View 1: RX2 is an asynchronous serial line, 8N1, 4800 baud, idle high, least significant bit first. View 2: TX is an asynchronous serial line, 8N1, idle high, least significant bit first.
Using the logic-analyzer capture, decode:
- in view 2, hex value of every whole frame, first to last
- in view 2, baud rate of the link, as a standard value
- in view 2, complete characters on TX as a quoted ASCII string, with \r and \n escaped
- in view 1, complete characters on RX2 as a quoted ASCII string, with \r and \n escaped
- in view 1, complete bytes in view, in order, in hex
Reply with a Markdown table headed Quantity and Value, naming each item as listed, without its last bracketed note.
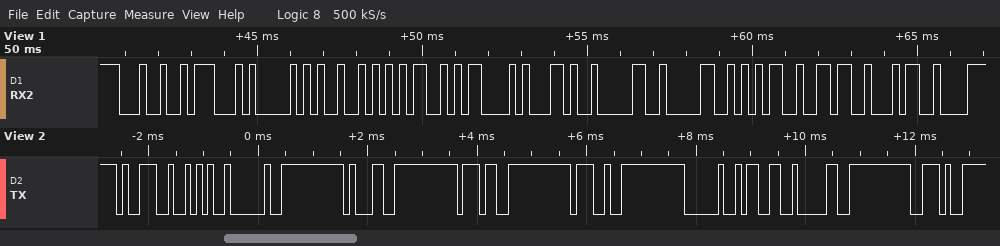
| Quantity | Value |
|---|---|
| in view 2, hex value of every whole frame, first to last | 39 2A 20 31 37 27 20 33 30 2E |
| in view 2, baud rate of the link, as a standard value | 9600 baud |
| in view 2, complete characters on TX as a quoted ASCII string, with \r and \n escaped | "9* 17' 30." |
| in view 1, complete characters on RX2 as a quoted ASCII string, with \r and \n escaped | "$GPRMC,00564" |
| in view 1, complete bytes in view, in order, in hex | 24 47 50 52 4D 43 2C 30 30 35 36 34 |
